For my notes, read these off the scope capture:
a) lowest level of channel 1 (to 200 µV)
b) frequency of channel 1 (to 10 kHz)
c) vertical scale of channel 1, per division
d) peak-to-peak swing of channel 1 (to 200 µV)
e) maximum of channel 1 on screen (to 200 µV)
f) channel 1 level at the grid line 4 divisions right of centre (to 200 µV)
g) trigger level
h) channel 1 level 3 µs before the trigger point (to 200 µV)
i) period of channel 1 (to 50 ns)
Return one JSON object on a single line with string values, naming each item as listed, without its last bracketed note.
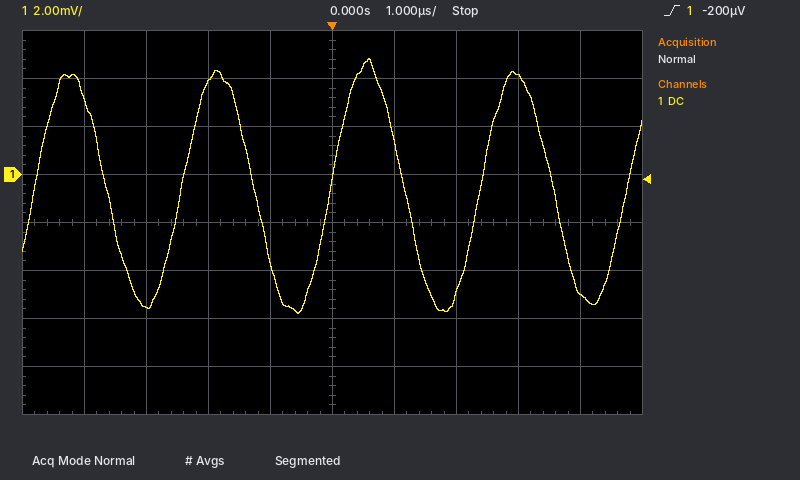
{"lowest level of channel 1": "-5.8 mV", "frequency of channel 1": "420 kHz", "vertical scale of channel 1, per division": "2 mV", "peak-to-peak swing of channel 1": "10.6 mV", "maximum of channel 1 on screen": "4.8 mV", "channel 1 level at the grid line 4 divisions right of centre": "-5.0 mV", "trigger level": "-200 µV", "channel 1 level 3 µs before the trigger point": "-5.6 mV", "period of channel 1": "2.40 µs"}
